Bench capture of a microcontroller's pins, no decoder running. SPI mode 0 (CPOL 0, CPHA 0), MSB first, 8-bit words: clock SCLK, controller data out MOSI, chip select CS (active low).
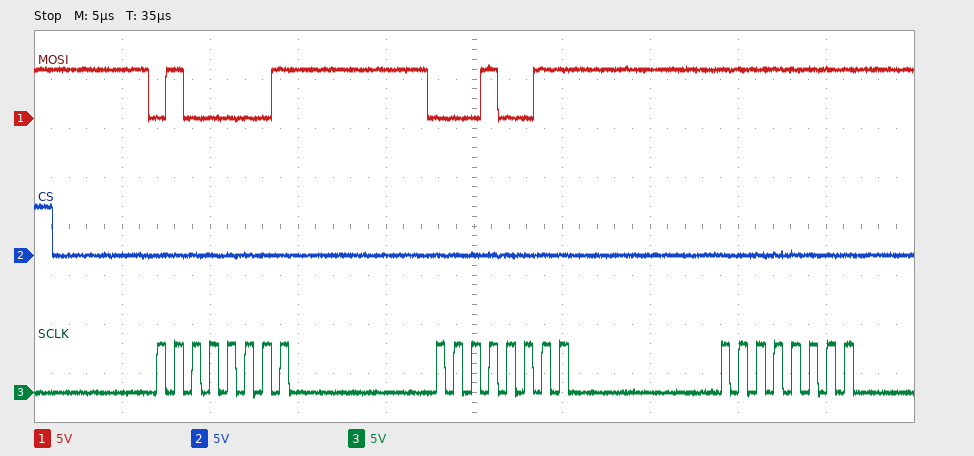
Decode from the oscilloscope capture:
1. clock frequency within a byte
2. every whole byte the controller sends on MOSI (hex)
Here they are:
1 MHz
41 13 FF
